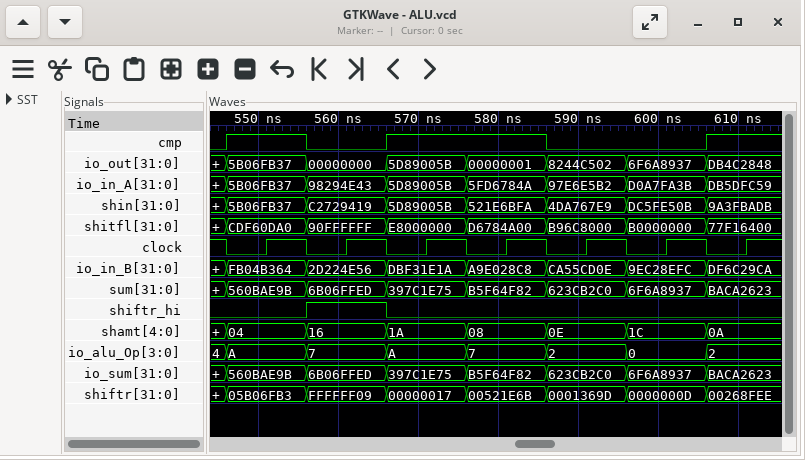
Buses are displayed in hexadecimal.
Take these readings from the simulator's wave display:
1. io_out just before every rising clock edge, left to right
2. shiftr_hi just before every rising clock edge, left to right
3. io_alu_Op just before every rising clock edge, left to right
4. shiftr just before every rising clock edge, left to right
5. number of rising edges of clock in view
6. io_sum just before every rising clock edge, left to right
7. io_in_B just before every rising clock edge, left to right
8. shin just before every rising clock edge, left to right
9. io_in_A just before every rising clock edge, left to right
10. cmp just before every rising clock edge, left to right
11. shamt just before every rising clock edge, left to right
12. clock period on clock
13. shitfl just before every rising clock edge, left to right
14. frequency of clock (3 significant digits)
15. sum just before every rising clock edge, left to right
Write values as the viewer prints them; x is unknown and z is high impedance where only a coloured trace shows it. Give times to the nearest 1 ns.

5B06FB37, 00000000, 5D89005B, 00000001, 8244C502, 6F6A8937, DB4C2848
0 1 0 0 0 0 0
A, 7, A, 7, 2, 0, 2
05B06FB3, FFFFFF09, 00000017, 00521E6B, 0001369D, 0000000D, 00268FEE
7
560BAE9B, 6B06FFED, 397C1E75, B5F64F82, 623CB2C0, 6F6A8937, BACA2623
FB04B364, 2D224E56, DBF31E1A, A9E028C8, CA55CD0E, 9EC28EFC, DF6C29CA
5B06FB37, C2729419, 5D89005B, 521E6BFA, 4DA767E9, DC5FE50B, 9A3FBADB
5B06FB37, 98294E43, 5D89005B, 5FD6784A, 97E6E5B2, D0A7FA3B, DB5DFC59
1 0 1 1 0 0 1
04, 16, 1A, 08, 0E, 1C, 0A
10 ns
CDF60DA0, 90FFFFFF, E8000000, D6784A00, B96C8000, B0000000, 77F16400
100 MHz
560BAE9B, 6B06FFED, 397C1E75, B5F64F82, 623CB2C0, 6F6A8937, BACA2623
